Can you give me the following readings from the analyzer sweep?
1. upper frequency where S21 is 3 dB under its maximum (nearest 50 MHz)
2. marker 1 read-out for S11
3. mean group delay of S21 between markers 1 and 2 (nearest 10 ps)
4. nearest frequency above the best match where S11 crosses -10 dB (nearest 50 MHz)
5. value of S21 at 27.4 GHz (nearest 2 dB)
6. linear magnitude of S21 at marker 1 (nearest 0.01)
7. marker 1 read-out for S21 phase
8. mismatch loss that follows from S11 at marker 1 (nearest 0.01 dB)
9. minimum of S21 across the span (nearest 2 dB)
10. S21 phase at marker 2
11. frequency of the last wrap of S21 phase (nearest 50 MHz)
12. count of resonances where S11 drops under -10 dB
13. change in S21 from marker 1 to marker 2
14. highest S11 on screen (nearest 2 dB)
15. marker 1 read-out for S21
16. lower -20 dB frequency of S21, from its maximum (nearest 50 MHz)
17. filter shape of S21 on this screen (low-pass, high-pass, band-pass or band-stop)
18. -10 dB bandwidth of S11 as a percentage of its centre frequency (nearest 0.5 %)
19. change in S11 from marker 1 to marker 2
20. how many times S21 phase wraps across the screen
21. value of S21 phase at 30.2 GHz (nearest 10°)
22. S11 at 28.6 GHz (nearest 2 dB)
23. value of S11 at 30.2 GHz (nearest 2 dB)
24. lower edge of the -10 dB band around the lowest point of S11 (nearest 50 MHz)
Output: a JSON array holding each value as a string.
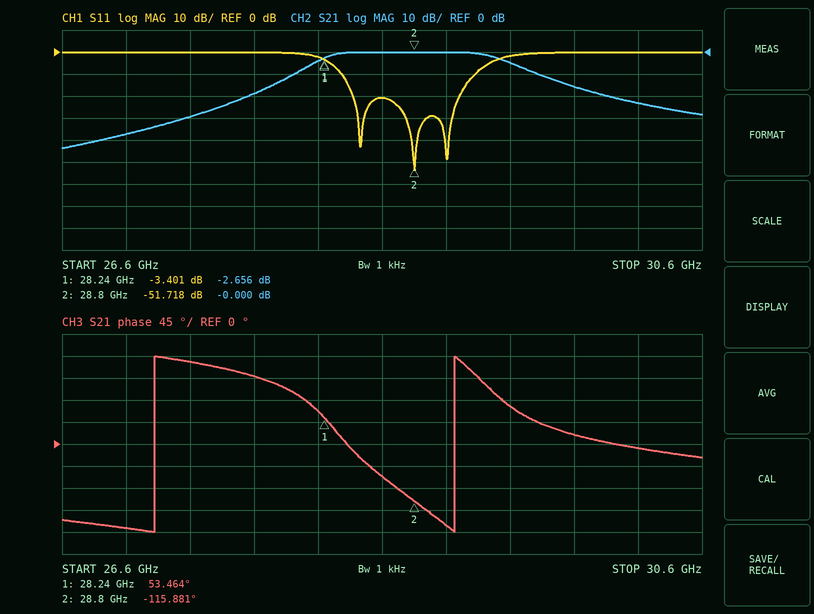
["29.35 GHz", "-3.401 dB", "840 ps", "29.20 GHz", "-30 dB", "0.74", "53.464°", "2.65 dB", "-44 dB", "-115.881°", "29.05 GHz", "3", "2.656 dB", "0 dB", "-2.656 dB", "27.75 GHz", "band-pass", "3.0 %", "-48.317 dB", "2", "-10°", "-20 dB", "0 dB", "28.35 GHz"]
